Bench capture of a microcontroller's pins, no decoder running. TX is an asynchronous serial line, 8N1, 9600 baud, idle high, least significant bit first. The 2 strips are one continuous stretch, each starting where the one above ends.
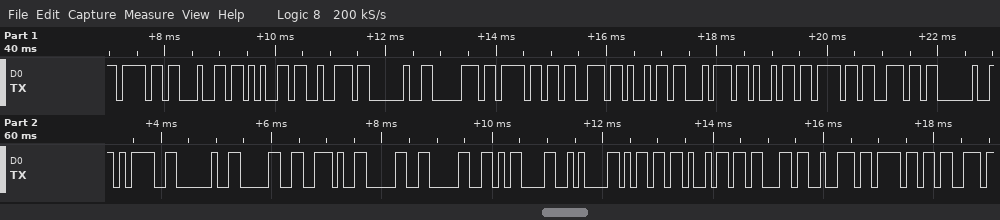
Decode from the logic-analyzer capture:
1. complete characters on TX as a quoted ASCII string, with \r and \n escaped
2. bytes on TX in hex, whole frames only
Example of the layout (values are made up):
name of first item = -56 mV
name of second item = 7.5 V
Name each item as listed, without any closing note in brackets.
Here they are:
complete characters on TX as a quoted ASCII string, with \r and \n escaped = "oder position = 0.00\r\nmicros"
bytes on TX in hex, whole frames only = 6F 64 65 72 20 70 6F 73 69 74 69 6F 6E 20 3D 20 30 2E 30 30 0D 0A 6D 69 63 72 6F 73
